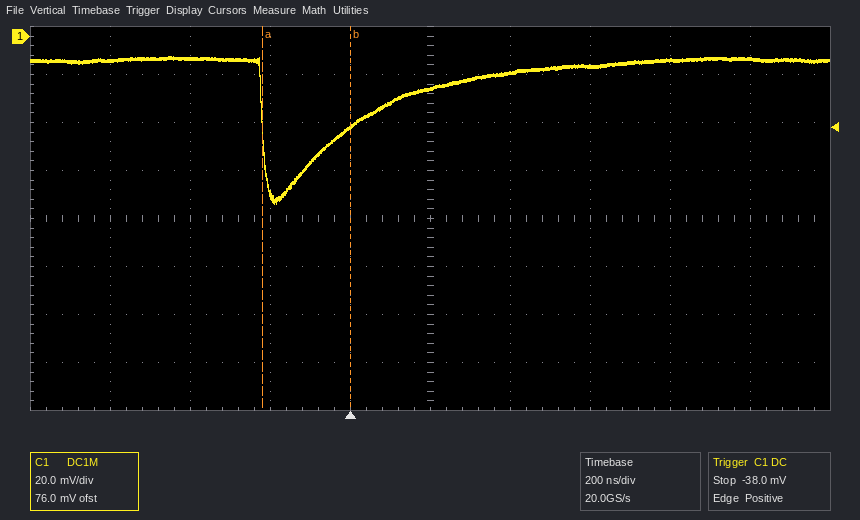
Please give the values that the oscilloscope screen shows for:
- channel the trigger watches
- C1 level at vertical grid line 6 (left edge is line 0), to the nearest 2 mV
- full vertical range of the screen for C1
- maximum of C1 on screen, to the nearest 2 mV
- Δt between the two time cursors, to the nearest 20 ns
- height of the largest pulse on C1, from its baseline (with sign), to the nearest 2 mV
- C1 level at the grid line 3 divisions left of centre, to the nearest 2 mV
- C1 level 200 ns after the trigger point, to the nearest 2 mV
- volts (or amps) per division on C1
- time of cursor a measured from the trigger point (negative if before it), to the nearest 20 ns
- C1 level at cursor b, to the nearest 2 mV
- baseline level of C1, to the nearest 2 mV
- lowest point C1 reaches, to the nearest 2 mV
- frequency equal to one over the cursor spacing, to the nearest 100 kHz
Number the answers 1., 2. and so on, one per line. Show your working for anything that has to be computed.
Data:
1. C1
2. -16 mV
3. 160 mV
4. -8 mV
5. 220 ns
6. -70 mV − (-10 mV) = -60 mV
7. -10 mV
8. -22 mV
9. 20 mV
10. -220 ns
11. -38 mV
12. -10 mV
13. -70 mV
14. 1 / 220 ns ≈ 4.5 MHz
